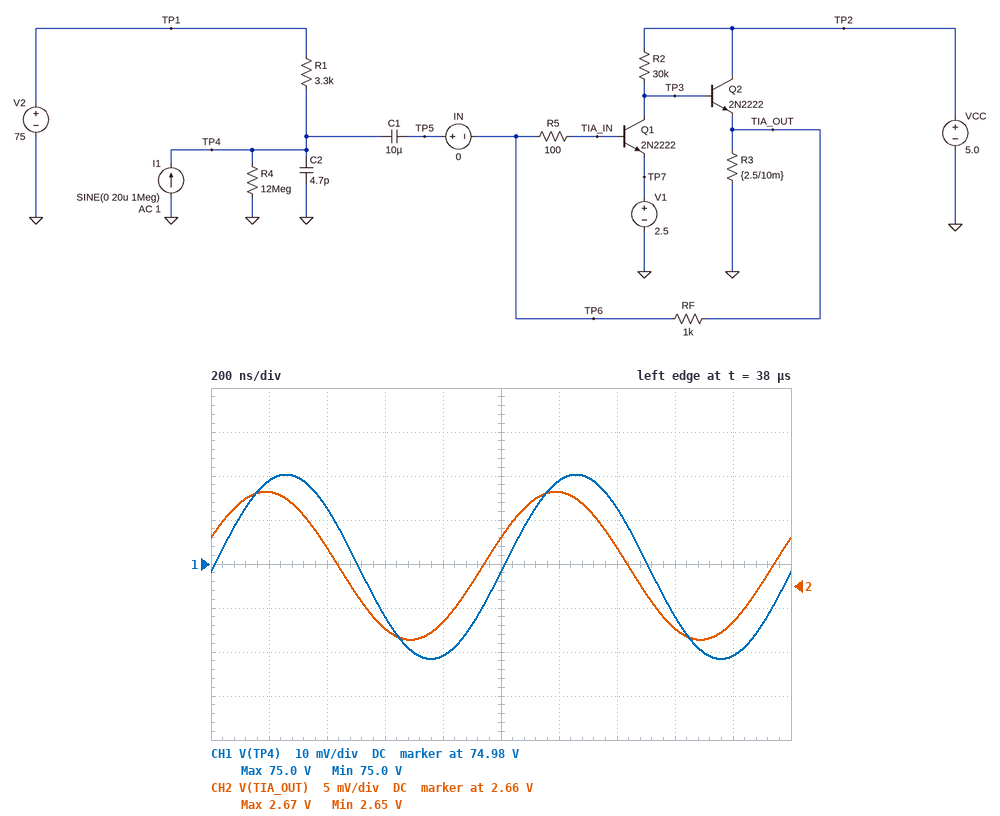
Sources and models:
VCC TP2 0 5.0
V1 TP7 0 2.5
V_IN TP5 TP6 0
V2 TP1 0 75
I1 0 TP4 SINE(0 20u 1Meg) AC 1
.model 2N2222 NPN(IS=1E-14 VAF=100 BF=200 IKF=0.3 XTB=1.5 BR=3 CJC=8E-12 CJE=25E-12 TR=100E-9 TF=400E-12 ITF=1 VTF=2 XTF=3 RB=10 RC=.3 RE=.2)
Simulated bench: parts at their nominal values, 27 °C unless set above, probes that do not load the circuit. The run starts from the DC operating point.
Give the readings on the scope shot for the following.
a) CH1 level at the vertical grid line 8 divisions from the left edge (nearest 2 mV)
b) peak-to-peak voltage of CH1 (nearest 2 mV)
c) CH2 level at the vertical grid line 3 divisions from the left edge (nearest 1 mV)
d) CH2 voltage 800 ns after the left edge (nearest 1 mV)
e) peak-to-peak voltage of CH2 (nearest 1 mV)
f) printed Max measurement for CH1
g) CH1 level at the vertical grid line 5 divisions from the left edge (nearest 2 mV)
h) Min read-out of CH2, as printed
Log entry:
74.968 V
42 mV
2.655 V
2.656 V
17 mV
75.0 V
74.978 V
2.65 V
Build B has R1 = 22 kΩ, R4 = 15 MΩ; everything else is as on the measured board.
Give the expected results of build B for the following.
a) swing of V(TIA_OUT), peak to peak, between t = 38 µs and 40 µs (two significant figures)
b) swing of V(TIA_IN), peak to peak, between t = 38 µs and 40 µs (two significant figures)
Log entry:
23 mV
57 mV
